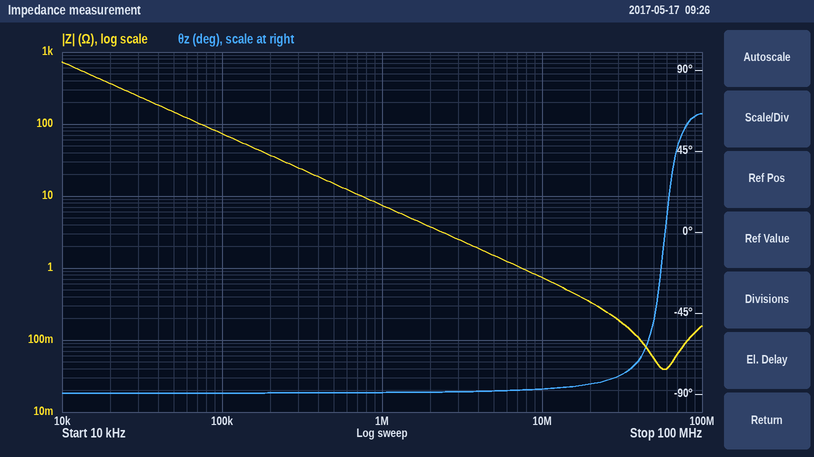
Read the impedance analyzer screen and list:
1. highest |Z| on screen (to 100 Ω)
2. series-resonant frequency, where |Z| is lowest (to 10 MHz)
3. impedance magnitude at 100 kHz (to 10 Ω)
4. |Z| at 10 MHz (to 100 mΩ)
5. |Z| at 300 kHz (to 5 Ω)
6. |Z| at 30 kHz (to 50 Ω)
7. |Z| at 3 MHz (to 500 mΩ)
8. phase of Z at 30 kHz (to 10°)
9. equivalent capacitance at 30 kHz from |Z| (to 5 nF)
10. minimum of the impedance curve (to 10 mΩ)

700 Ω
60 MHz
70 Ω
700 mΩ
25 Ω
250 Ω
2.5 Ω
-90°
20 nF
40 mΩ
